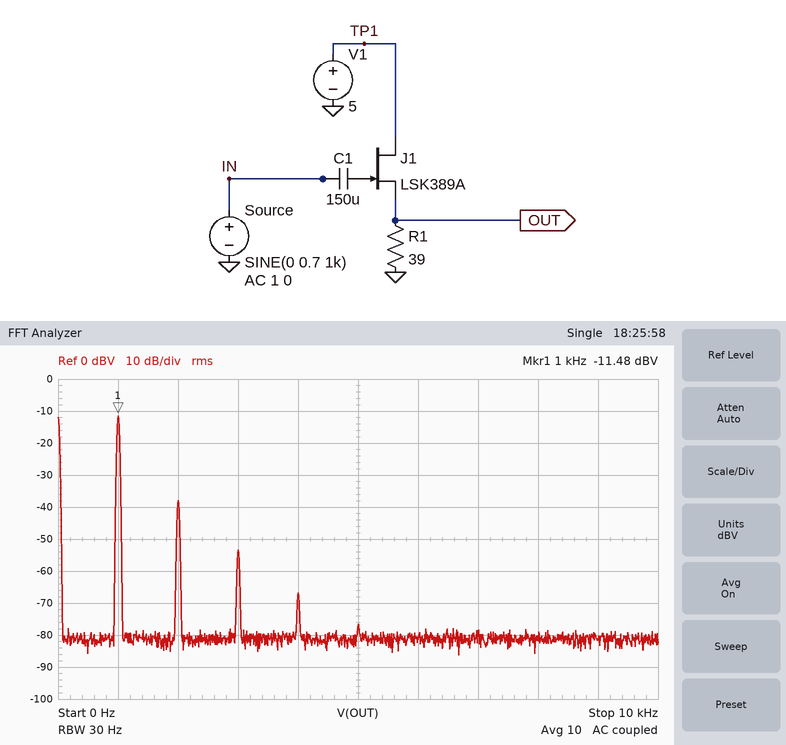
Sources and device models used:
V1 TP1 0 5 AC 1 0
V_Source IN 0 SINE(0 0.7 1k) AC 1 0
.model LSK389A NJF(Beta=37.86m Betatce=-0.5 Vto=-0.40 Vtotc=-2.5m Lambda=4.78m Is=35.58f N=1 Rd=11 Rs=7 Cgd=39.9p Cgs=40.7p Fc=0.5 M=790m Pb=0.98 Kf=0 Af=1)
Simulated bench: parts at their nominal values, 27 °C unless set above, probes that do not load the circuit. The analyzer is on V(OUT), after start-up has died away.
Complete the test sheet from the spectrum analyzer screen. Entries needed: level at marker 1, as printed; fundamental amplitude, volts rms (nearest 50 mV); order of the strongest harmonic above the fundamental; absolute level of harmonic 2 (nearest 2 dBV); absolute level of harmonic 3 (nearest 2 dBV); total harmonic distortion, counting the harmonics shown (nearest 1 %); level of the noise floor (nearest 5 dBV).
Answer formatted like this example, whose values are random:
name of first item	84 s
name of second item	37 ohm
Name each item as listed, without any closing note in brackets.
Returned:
level at marker 1, as printed	-11.48 dBV
fundamental amplitude, volts rms	250 mV
order of the strongest harmonic above the fundamental	2
absolute level of harmonic 2	-38 dBV
absolute level of harmonic 3	-54 dBV
total harmonic distortion, counting the harmonics shown	5 %
level of the noise floor	-80 dBV
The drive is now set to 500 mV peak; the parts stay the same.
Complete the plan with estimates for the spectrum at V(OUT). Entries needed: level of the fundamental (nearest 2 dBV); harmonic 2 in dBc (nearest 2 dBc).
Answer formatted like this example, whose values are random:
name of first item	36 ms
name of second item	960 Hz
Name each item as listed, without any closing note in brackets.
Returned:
level of the fundamental	-14 dBV
harmonic 2 in dBc	-30 dBc
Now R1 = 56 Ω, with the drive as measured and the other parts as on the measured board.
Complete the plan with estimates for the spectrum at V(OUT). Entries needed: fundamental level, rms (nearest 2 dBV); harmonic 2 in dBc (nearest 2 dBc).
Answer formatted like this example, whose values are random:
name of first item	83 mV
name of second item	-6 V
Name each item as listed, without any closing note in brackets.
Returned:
fundamental level, rms	-10 dBV
harmonic 2 in dBc	-30 dBc
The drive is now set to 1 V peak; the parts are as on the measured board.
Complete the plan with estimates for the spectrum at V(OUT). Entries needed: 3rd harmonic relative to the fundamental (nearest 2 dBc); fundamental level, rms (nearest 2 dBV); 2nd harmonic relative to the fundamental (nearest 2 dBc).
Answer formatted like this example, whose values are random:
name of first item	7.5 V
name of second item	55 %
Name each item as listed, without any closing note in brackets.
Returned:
3rd harmonic relative to the fundamental	-32 dBc
fundamental level, rms	-8 dBV
2nd harmonic relative to the fundamental	-22 dBc
